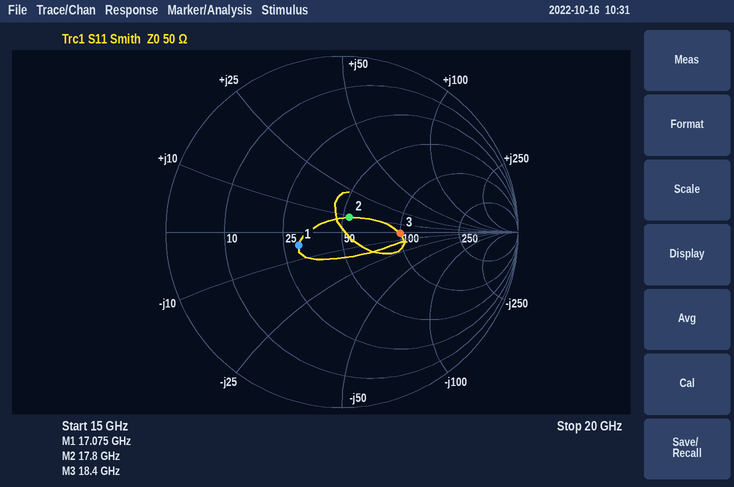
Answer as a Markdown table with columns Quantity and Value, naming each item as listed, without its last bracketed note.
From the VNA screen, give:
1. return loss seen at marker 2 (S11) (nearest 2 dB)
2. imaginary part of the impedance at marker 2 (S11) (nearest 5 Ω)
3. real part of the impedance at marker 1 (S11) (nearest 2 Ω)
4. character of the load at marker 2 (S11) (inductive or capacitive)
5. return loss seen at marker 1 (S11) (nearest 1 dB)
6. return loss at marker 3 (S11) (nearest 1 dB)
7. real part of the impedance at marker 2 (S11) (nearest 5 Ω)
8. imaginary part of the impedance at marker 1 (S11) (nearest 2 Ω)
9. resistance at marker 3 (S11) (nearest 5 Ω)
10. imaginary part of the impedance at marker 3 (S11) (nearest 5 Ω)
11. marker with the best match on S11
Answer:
| Quantity | Value |
|---|---|
| return loss seen at marker 2 (S11) | 20 dB |
| imaginary part of the impedance at marker 2 (S11) | +10 Ω |
| real part of the impedance at marker 1 (S11) | 30 Ω |
| character of the load at marker 2 (S11) | inductive |
| return loss seen at marker 1 (S11) | 12 dB |
| return loss at marker 3 (S11) | 10 dB |
| real part of the impedance at marker 2 (S11) | 55 Ω |
| imaginary part of the impedance at marker 1 (S11) | -4 Ω |
| resistance at marker 3 (S11) | 100 Ω |
| imaginary part of the impedance at marker 3 (S11) | 0 Ω |
| marker with the best match on S11 | marker 2 |
